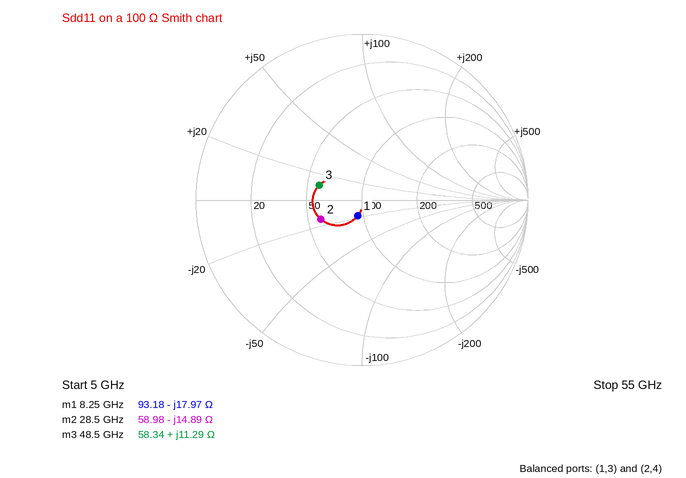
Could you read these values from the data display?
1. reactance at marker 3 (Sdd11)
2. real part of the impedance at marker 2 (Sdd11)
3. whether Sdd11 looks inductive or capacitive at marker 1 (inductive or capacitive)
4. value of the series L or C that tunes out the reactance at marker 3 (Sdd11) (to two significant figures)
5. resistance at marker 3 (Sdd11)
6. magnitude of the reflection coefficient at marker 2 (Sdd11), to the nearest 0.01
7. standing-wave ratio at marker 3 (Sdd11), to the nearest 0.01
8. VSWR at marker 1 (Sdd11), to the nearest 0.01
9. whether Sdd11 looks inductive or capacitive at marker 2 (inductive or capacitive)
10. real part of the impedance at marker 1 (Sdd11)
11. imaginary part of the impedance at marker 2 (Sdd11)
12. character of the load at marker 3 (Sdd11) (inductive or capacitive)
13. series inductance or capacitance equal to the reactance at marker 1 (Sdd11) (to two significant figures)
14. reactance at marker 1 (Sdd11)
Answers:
+11.29 Ω
58.98 Ω
capacitive
290 fF
58.34 Ω
0.27
1.75
1.22
capacitive
93.18 Ω
-14.89 Ω
inductive
1.1 pF
-17.97 Ω
